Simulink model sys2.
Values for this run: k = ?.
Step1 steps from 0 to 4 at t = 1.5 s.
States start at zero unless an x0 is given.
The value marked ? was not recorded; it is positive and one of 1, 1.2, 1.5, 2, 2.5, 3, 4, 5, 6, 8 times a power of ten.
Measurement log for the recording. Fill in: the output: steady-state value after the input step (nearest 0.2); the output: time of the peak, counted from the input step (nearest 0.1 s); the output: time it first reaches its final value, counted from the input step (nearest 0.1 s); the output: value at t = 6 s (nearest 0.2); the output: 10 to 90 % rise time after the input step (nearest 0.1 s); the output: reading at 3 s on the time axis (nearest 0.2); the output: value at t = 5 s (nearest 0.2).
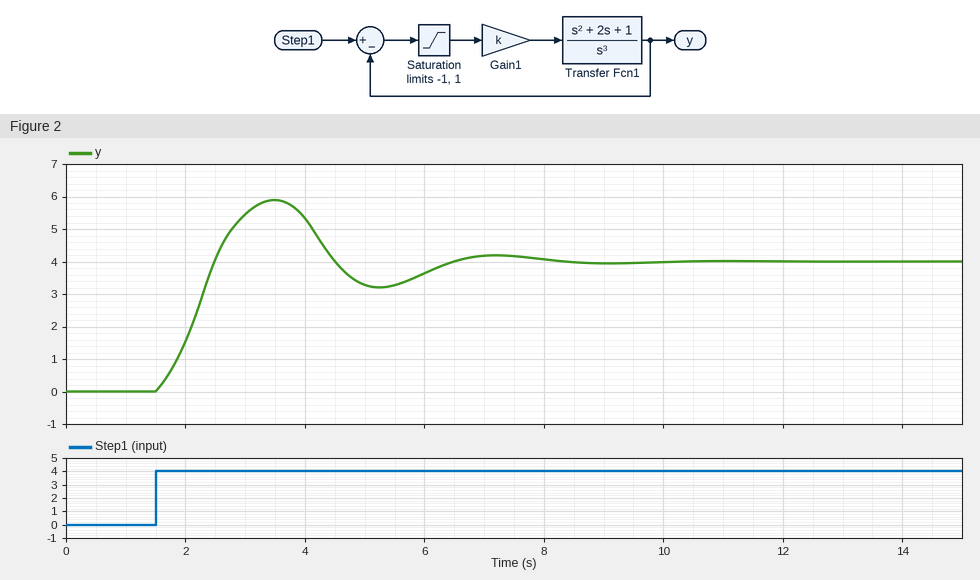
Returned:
4.0
2.0 s
1.0 s
3.6
0.7 s
5.4
3.2
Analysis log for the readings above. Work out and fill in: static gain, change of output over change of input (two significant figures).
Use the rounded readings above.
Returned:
1.0
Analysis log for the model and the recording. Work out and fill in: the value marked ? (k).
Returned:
2
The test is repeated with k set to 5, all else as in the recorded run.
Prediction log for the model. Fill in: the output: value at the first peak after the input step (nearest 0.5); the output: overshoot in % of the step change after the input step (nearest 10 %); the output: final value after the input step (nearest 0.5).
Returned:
5.0
20 %
4.0
